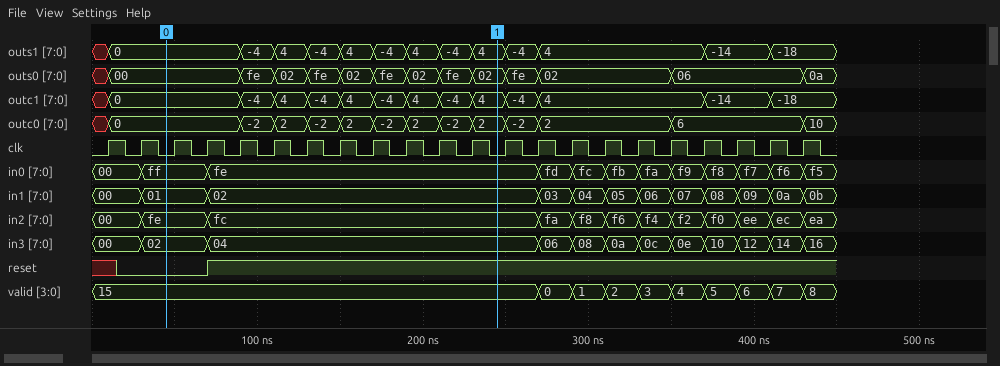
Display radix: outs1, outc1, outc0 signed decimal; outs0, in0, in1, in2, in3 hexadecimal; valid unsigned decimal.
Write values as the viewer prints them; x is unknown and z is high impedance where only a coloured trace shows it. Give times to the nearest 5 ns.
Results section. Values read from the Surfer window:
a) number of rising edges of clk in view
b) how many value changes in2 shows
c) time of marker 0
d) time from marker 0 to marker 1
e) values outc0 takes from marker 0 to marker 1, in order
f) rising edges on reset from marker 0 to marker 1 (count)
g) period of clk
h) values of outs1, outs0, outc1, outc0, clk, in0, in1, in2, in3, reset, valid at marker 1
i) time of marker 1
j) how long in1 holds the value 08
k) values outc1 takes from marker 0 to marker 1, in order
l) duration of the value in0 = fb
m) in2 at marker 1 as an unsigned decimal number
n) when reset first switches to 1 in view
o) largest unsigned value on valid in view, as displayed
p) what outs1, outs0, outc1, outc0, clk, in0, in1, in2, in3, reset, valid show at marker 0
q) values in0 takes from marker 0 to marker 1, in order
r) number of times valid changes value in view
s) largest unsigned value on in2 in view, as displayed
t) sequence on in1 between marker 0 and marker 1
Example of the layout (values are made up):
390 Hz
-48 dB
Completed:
22
11
45 ns
200 ns
0, -2, 2, -2, 2, -2, 2, -2, 2
1
20 ns
outs1=4, outs0=02, outc1=4, outc0=2, clk=0, in0=fe, in1=02, in2=fc, in3=04, reset=1, valid=15
245 ns
20 ns
0, -4, 4, -4, 4, -4, 4, -4, 4
20 ns
252
70 ns
15
outs1=0, outs0=00, outc1=0, outc0=0, clk=0, in0=ff, in1=01, in2=fe, in3=02, reset=0, valid=15
ff, fe
9
fe
01, 02
